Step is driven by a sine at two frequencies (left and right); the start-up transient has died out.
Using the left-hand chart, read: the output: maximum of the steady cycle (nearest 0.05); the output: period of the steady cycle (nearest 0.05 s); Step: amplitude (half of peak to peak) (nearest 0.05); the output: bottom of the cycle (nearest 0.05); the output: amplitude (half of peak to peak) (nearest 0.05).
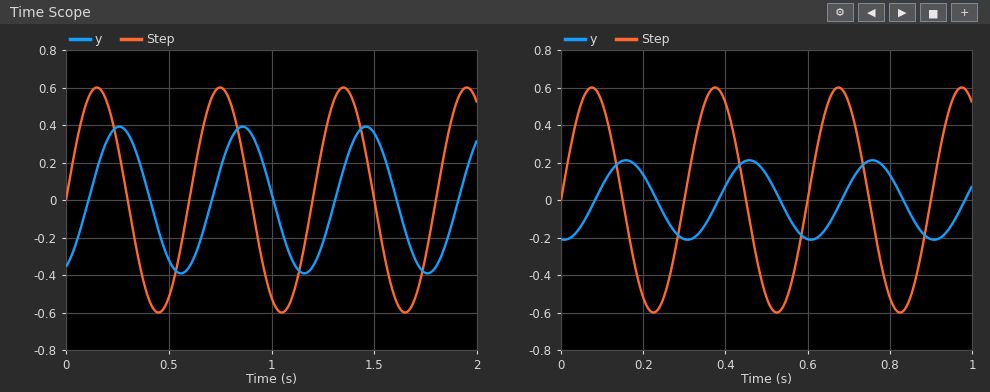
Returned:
0.40
0.60 s
0.60
-0.40
0.40
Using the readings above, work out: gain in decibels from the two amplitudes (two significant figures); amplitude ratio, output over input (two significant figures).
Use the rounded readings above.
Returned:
-3.5 dB
0.67
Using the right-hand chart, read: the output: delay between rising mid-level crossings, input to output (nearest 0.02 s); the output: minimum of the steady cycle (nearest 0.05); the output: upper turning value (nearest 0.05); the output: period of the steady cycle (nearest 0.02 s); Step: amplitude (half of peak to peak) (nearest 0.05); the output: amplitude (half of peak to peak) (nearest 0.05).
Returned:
0.08 s
-0.20
0.20
0.30 s
0.60
0.20
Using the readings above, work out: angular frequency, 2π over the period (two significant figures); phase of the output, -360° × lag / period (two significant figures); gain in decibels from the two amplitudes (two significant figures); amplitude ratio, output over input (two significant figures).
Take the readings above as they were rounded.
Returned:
21 rad/s
-96°
-9.5 dB
0.33
